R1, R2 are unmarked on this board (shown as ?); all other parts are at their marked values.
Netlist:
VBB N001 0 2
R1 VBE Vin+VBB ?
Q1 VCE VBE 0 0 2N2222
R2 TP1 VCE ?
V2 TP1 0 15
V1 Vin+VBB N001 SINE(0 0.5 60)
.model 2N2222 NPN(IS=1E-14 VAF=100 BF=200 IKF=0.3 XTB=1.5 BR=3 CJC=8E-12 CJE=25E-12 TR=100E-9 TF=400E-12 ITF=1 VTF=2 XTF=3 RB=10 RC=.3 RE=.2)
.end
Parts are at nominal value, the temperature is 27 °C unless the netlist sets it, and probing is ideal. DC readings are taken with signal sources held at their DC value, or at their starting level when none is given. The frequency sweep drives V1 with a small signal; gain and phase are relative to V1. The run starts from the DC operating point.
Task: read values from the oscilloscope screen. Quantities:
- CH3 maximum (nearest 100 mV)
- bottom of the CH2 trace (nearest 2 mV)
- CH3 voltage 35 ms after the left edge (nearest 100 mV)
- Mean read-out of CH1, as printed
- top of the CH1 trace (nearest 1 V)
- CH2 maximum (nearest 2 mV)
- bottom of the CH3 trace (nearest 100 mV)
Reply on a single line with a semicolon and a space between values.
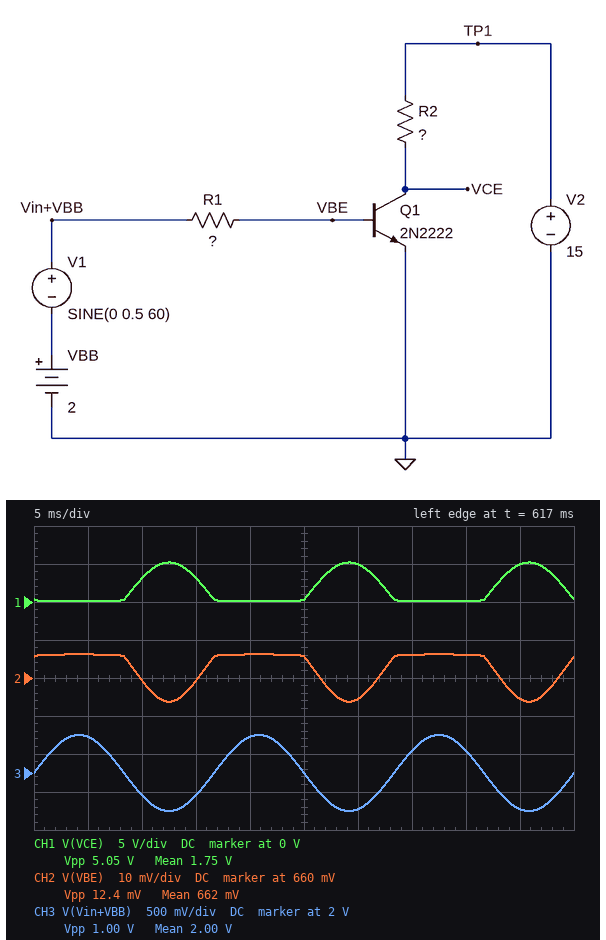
2.5 V; 654 mV; 2.3 V; 1.75 V; 5 V; 666 mV; 1.5 V
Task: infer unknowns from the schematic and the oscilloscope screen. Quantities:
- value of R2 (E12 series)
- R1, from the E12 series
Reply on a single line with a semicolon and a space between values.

10 kΩ; 180 kΩ
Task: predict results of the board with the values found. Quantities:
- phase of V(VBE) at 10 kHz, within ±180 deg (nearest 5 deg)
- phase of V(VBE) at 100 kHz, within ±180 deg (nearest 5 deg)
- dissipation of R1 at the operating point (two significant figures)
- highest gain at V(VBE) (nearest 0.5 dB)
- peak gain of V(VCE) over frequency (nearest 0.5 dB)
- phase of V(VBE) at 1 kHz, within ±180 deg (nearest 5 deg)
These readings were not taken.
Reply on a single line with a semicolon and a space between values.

-40 deg; -80 deg; 9.9 µW; -36.0 dB; 17.5 dB; -5 deg
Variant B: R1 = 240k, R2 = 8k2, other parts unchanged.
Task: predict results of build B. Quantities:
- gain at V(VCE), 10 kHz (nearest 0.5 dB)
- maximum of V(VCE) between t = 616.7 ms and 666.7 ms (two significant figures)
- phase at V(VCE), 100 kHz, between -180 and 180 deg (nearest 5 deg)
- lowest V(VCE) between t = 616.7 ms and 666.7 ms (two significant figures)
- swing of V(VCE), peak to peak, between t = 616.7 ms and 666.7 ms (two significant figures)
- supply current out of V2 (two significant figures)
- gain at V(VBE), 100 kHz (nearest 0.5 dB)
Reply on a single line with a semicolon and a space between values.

15.5 dB; 8.7 V; 105 deg; 2.3 V; 6.4 V; 1.2 mA; -47.0 dB
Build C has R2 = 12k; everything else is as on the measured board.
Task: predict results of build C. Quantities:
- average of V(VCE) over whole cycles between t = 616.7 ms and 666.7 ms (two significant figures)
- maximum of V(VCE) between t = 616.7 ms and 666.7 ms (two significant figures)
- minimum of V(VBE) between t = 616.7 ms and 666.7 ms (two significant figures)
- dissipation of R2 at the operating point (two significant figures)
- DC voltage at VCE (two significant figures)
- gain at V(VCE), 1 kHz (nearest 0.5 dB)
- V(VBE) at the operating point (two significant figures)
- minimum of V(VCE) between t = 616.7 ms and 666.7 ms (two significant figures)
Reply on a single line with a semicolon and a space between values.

910 mV; 3.4 V; 650 mV; 18 mW; 150 mV; -18.5 dB; 660 mV; 120 mV
